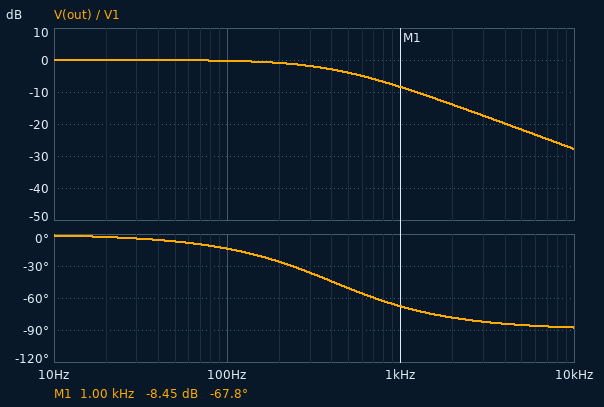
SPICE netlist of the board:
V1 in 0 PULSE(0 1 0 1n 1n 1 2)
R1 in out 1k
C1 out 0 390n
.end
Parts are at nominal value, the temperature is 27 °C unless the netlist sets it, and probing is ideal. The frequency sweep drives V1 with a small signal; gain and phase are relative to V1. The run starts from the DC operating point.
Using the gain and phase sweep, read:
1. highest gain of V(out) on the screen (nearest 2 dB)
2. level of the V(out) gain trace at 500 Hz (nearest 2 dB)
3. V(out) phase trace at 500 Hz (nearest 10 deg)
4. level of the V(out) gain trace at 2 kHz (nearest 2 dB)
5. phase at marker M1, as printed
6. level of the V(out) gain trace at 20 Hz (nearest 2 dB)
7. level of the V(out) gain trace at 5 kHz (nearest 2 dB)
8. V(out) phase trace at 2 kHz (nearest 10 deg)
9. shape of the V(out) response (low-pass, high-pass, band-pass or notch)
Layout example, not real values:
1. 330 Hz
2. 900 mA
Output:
1. 0 dB
2. -4 dB
3. -50 deg
4. -14 dB
5. -67.8 deg
6. 0 dB
7. -22 dB
8. -80 deg
9. low-pass
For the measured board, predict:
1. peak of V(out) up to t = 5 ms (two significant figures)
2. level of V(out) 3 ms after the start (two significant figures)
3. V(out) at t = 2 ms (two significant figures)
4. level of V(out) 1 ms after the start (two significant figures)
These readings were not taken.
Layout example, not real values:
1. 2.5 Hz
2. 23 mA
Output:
1. 1.0 V
2. 1.0 V
3. 990 mV
4. 920 mV
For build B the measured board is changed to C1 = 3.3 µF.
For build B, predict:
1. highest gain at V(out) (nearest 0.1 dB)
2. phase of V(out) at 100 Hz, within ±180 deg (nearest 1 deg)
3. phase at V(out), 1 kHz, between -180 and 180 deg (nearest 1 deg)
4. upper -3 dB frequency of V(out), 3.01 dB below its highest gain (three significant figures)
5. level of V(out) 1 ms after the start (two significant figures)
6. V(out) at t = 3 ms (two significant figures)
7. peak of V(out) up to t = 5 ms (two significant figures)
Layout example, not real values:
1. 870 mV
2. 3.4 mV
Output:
1. 0 dB
2. -64 deg
3. -87 deg
4. 48.2 Hz
5. 260 mV
6. 600 mV
7. 780 mV
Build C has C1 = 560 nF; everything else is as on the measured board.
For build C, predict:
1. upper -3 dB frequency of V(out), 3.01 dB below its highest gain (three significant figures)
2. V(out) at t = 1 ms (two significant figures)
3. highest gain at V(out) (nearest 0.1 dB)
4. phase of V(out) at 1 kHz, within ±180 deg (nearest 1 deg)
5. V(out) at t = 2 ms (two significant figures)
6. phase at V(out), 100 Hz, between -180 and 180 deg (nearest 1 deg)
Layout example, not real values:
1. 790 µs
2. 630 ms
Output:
1. 284 Hz
2. 830 mV
3. 0 dB
4. -74 deg
5. 970 mV
6. -19 deg
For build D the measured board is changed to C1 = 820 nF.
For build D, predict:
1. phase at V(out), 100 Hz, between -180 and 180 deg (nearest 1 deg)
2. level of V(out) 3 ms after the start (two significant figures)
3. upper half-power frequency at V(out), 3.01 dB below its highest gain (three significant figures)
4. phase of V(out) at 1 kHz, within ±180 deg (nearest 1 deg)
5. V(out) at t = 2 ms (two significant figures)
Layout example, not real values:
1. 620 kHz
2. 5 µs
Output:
1. -27 deg
2. 970 mV
3. 194 Hz
4. -79 deg
5. 910 mV
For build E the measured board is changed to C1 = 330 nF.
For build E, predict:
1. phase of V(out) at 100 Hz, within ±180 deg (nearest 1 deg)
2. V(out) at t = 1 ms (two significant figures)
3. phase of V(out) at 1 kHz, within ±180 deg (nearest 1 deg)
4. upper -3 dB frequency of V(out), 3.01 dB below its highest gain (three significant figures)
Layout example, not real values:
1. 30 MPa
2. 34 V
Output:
1. -12 deg
2. 950 mV
3. -64 deg
4. 482 Hz
